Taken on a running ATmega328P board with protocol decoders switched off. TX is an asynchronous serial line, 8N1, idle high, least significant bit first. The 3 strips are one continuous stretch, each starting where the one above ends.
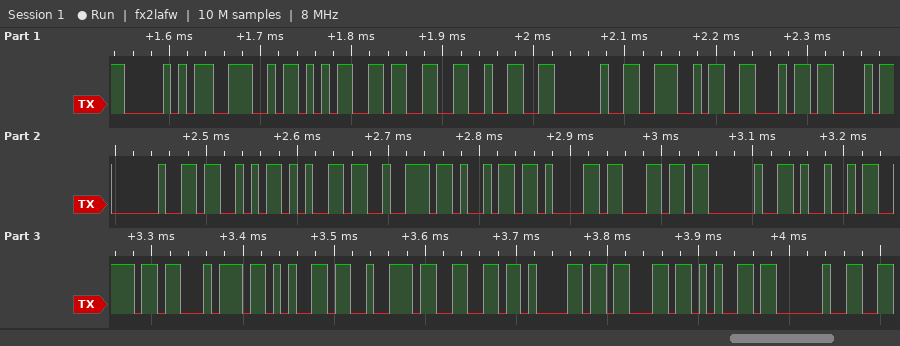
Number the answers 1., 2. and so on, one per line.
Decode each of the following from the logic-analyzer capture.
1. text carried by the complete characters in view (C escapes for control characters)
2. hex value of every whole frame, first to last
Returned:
1. "PN532 NFC Serial Interface "
2. 50 4E 35 33 32 20 4E 46 43 20 53 65 72 69 61 6C 20 49 6E 74 65 72 66 61 63 65 20
